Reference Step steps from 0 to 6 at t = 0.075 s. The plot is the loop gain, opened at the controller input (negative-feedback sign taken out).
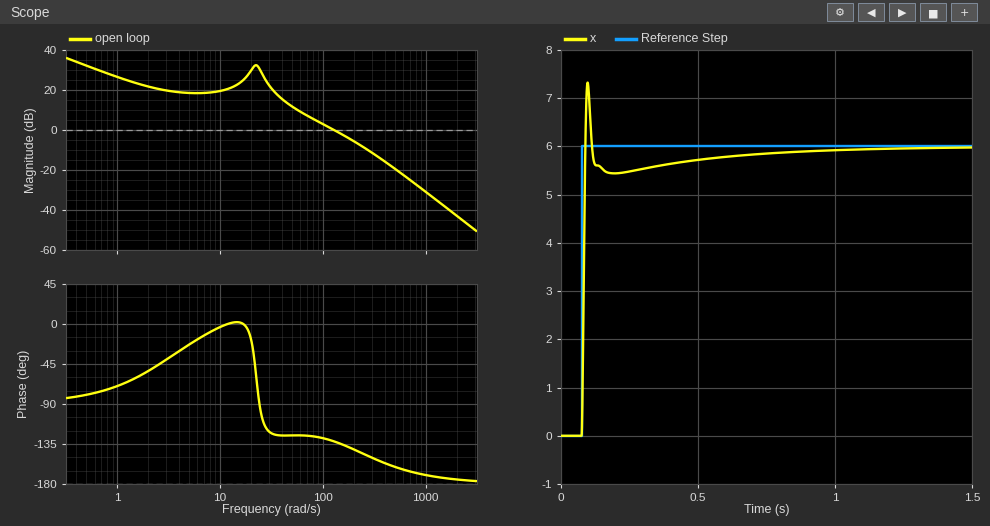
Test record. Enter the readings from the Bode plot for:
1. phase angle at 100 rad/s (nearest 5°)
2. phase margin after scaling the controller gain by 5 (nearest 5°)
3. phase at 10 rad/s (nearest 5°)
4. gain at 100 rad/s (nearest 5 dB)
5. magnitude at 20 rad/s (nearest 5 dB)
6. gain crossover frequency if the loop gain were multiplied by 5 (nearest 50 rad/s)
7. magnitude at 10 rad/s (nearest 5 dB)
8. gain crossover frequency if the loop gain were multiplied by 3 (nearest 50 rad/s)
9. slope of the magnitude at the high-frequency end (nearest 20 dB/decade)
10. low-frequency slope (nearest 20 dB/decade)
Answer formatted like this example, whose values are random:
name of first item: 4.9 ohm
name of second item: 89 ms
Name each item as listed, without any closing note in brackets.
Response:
phase angle at 100 rad/s: -130°
phase margin after scaling the controller gain by 5: 25°
phase at 10 rad/s: -5°
gain at 100 rad/s: 5 dB
magnitude at 20 rad/s: 30 dB
gain crossover frequency if the loop gain were multiplied by 5: 350 rad/s
magnitude at 10 rad/s: 20 dB
gain crossover frequency if the loop gain were multiplied by 3: 250 rad/s
slope of the magnitude at the high-frequency end: -40 dB/decade
low-frequency slope: -20 dB/decade
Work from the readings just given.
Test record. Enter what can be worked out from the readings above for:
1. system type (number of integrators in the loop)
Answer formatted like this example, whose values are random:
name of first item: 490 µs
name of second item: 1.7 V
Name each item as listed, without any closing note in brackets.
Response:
system type: 1
